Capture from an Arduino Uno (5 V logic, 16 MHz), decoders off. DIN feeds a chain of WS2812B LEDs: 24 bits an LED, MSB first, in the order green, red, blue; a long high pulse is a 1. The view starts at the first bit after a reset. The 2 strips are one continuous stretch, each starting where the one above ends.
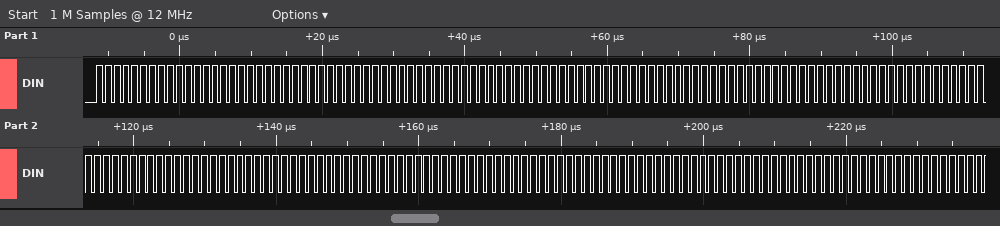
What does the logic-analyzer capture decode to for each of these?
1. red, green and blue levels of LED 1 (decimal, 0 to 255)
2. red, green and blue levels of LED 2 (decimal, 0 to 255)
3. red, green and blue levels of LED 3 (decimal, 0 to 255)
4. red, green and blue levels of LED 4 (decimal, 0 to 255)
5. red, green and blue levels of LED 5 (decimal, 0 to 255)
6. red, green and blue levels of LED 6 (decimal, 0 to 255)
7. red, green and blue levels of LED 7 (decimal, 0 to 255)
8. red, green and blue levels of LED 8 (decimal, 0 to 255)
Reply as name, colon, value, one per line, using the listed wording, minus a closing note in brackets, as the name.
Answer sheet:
red, green and blue levels of LED 1: 255, 255, 255
red, green and blue levels of LED 2: 255, 255, 255
red, green and blue levels of LED 3: 255, 255, 255
red, green and blue levels of LED 4: 255, 255, 255
red, green and blue levels of LED 5: 255, 255, 255
red, green and blue levels of LED 6: 255, 255, 255
red, green and blue levels of LED 7: 255, 255, 255
red, green and blue levels of LED 8: 255, 255, 255
